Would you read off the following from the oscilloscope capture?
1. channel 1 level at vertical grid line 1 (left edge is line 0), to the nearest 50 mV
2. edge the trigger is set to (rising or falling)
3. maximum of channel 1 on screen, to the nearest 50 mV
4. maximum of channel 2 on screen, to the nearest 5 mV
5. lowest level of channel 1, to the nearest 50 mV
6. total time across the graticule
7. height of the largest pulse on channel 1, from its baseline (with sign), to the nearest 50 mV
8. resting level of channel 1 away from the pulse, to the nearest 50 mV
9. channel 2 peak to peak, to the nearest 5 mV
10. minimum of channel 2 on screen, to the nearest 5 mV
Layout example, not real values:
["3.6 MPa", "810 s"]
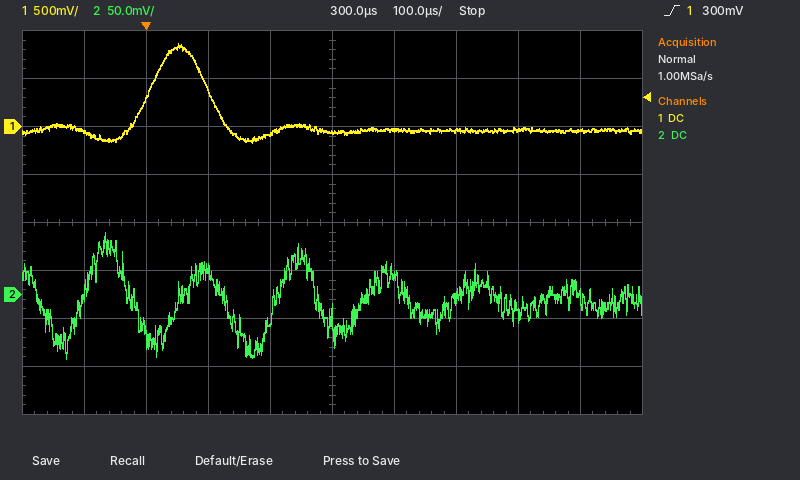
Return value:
["-50 mV", "rising", "850 mV", "65 mV", "-150 mV", "1 ms", "+900 mV", "-50 mV", "130 mV", "-65 mV"]
